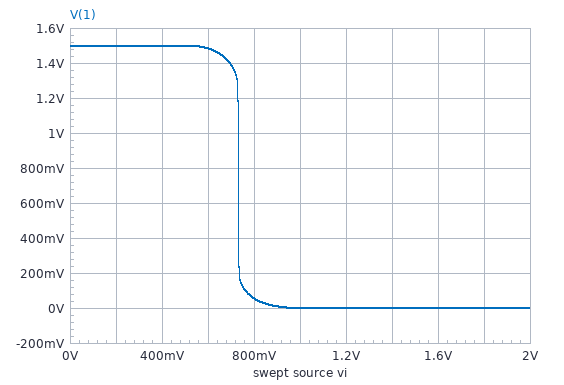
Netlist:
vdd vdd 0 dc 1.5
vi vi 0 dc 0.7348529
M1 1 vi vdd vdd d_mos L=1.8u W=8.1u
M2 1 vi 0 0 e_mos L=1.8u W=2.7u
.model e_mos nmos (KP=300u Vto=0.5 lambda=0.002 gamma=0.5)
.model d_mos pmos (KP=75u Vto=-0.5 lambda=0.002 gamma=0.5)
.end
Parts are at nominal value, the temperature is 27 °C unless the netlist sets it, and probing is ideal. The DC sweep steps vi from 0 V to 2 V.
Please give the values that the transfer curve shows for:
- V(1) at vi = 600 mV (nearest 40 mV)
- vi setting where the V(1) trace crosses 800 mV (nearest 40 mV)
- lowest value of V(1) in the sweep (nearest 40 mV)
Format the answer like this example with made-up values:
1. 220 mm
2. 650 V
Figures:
1. 1.48 V
2. 720 mV
3. 0 V
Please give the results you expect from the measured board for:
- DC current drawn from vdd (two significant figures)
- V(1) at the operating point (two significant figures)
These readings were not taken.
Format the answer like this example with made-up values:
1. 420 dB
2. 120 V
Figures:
1. 12 µA
2. 190 mV
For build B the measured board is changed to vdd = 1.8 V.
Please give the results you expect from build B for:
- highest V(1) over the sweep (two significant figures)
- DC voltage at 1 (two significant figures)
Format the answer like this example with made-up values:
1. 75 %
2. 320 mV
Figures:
1. 1.8 V
2. 1.7 V
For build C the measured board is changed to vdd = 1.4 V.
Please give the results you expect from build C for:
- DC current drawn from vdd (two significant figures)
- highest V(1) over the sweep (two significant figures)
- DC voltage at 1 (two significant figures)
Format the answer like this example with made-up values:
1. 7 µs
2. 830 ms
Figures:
1. 4.6 µA
2. 1.4 V
3. 49 mV
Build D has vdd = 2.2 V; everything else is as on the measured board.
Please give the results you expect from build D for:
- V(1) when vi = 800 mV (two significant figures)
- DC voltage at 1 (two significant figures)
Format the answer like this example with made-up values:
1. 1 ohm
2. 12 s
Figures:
1. 2.1 V
2. 2.2 V
